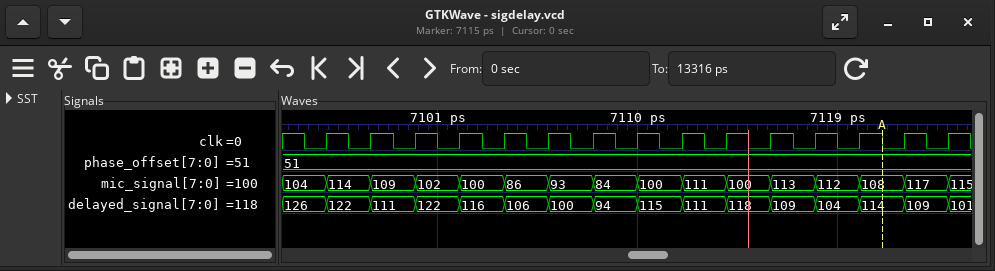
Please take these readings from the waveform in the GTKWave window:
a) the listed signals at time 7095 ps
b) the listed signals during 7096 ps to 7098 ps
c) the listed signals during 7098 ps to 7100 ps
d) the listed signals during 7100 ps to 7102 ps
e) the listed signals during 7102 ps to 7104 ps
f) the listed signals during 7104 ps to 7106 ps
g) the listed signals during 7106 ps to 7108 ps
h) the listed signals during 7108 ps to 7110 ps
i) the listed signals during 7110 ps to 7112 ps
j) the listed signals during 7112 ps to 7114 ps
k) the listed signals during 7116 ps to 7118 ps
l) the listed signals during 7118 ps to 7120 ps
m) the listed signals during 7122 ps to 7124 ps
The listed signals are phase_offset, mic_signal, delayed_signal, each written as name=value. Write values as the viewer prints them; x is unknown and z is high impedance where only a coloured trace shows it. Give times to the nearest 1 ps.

phase_offset=51, mic_signal=104, delayed_signal=126
phase_offset=51, mic_signal=114, delayed_signal=122
phase_offset=51, mic_signal=109, delayed_signal=111
phase_offset=51, mic_signal=102, delayed_signal=122
phase_offset=51, mic_signal=100, delayed_signal=116
phase_offset=51, mic_signal=86, delayed_signal=106
phase_offset=51, mic_signal=93, delayed_signal=100
phase_offset=51, mic_signal=84, delayed_signal=94
phase_offset=51, mic_signal=100, delayed_signal=115
phase_offset=51, mic_signal=111, delayed_signal=111
phase_offset=51, mic_signal=113, delayed_signal=109
phase_offset=51, mic_signal=112, delayed_signal=104
phase_offset=51, mic_signal=117, delayed_signal=109
